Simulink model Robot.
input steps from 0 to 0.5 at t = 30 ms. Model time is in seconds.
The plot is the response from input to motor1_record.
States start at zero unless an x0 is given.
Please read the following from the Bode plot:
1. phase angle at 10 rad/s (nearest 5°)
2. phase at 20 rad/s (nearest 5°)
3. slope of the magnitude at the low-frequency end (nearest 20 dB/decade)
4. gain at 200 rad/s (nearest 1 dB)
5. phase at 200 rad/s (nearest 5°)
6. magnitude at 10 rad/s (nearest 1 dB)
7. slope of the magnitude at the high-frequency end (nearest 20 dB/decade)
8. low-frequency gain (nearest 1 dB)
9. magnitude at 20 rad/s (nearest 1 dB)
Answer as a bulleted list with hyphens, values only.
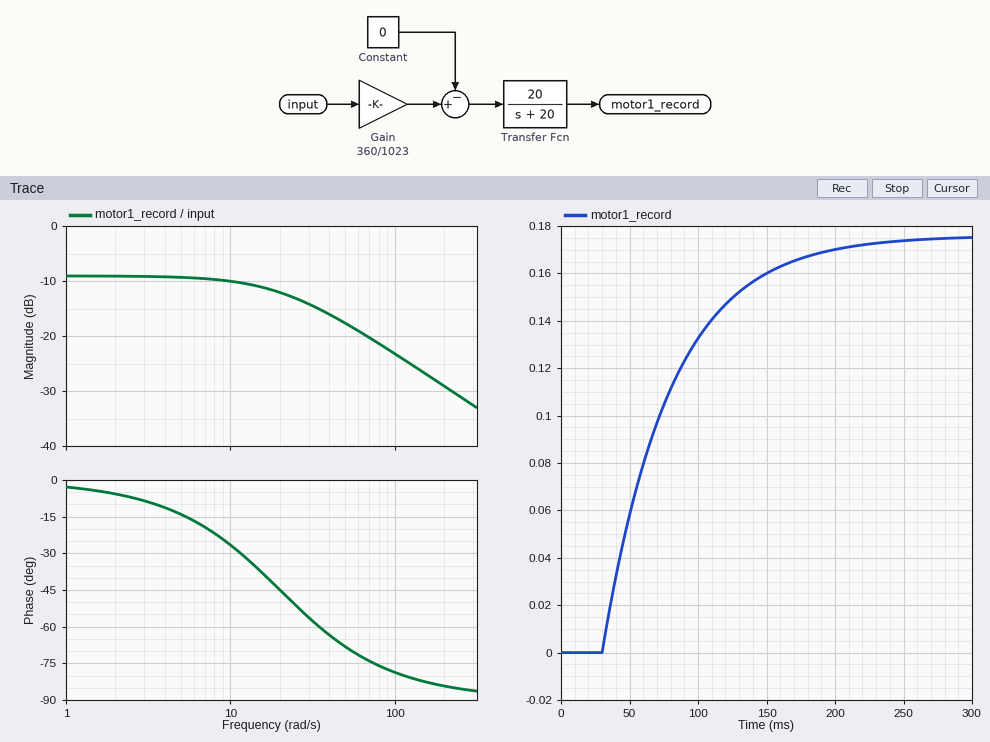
- -25°
- -45°
- 0 dB/decade
- -29 dB
- -85°
- -10 dB
- -20 dB/decade
- -9 dB
- -12 dB
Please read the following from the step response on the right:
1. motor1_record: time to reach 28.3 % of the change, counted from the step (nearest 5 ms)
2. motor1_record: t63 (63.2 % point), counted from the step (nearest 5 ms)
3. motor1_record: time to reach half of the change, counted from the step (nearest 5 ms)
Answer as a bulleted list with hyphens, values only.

- 15 ms
- 50 ms
- 35 ms
